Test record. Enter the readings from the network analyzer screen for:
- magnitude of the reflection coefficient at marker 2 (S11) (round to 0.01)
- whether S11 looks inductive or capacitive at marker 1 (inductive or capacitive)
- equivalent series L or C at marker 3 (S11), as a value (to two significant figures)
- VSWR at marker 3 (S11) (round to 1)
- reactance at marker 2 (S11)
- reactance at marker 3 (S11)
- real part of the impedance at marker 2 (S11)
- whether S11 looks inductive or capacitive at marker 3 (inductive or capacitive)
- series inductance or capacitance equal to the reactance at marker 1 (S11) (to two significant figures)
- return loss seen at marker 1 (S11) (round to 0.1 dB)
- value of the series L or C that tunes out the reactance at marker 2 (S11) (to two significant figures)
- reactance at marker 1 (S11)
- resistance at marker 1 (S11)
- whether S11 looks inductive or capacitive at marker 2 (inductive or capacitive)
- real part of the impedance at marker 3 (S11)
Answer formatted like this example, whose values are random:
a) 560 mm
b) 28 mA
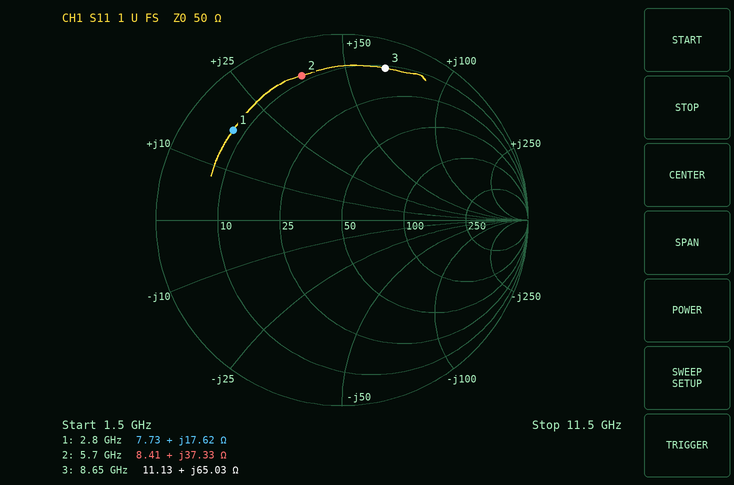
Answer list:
a) 0.81
b) inductive
c) 1.2 nH
d) 12
e) +37.33 Ω
f) +65.03 Ω
g) 8.41 Ω
h) inductive
i) 1.0 nH
j) 2.4 dB
k) 750 fF
l) +17.62 Ω
m) 7.73 Ω
n) inductive
o) 11.13 Ω
